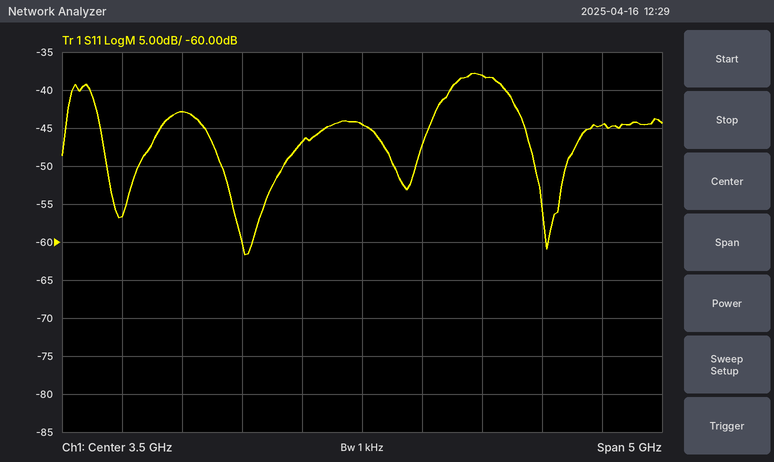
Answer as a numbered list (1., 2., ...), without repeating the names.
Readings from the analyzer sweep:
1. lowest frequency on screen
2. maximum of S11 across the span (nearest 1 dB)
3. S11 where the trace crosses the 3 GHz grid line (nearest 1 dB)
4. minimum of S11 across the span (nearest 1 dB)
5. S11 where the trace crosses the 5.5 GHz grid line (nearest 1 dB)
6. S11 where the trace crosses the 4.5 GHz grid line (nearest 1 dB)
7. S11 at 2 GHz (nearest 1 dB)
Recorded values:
1. 1 GHz
2. -38 dB
3. -47 dB
4. -62 dB
5. -45 dB
6. -38 dB
7. -43 dB
